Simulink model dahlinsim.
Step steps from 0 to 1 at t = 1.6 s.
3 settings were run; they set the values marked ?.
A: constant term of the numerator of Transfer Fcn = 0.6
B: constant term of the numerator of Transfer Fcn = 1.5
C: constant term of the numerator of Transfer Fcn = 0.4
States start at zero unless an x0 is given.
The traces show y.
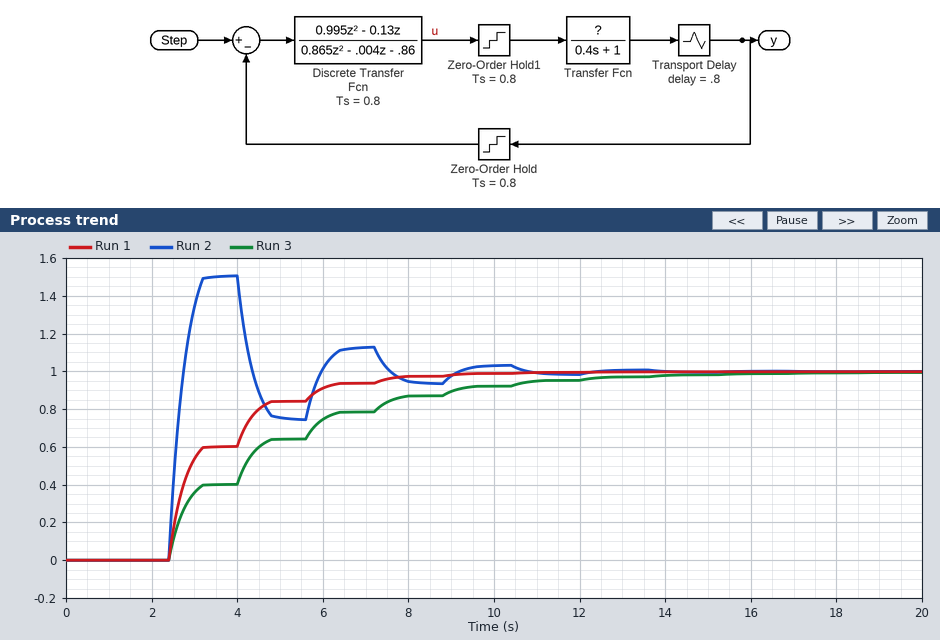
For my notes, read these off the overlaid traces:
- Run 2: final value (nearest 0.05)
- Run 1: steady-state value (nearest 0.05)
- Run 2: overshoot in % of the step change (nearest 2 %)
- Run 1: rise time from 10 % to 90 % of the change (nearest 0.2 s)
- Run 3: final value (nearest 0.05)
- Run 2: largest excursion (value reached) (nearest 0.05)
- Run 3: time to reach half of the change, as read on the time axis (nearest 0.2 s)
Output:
1.00
1.00
50 %
3.4 s
1.00
1.50
4.2 s
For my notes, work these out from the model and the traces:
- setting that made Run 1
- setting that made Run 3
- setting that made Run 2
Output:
A
C
B
